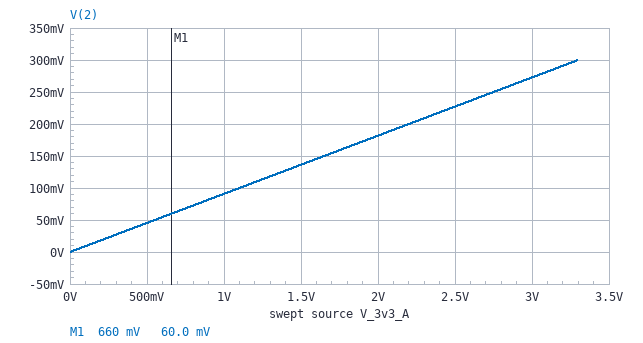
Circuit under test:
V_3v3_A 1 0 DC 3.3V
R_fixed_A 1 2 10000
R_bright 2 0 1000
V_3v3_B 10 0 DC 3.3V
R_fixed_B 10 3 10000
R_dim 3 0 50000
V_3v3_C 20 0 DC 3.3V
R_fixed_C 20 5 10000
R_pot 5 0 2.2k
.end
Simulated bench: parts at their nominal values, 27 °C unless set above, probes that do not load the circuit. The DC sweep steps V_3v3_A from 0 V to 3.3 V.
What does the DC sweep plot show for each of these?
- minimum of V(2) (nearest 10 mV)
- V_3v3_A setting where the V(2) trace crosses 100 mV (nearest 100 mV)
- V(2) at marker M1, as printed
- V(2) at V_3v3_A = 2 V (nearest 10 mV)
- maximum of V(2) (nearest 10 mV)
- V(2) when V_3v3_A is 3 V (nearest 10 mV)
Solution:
0 V
1.1 V
60.0 mV
180 mV
300 mV
270 mV
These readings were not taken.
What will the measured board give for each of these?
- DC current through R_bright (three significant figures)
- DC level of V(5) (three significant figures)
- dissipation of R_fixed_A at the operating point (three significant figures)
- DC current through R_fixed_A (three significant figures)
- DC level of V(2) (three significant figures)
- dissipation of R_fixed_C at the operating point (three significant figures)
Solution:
300 µA
595 mV
900 µW
300 µA
300 mV
732 µW
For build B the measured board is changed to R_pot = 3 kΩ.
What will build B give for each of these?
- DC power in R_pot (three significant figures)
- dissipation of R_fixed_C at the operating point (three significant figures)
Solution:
193 µW
644 µW
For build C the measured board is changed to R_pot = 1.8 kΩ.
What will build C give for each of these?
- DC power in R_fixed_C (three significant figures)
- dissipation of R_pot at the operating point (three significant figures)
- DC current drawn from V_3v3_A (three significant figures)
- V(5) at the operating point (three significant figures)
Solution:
782 µW
141 µW
300 µA
503 mV
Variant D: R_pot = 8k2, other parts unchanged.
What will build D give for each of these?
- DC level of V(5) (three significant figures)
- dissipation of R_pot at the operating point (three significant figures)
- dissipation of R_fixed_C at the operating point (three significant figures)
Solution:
1.49 V
270 µW
329 µW
